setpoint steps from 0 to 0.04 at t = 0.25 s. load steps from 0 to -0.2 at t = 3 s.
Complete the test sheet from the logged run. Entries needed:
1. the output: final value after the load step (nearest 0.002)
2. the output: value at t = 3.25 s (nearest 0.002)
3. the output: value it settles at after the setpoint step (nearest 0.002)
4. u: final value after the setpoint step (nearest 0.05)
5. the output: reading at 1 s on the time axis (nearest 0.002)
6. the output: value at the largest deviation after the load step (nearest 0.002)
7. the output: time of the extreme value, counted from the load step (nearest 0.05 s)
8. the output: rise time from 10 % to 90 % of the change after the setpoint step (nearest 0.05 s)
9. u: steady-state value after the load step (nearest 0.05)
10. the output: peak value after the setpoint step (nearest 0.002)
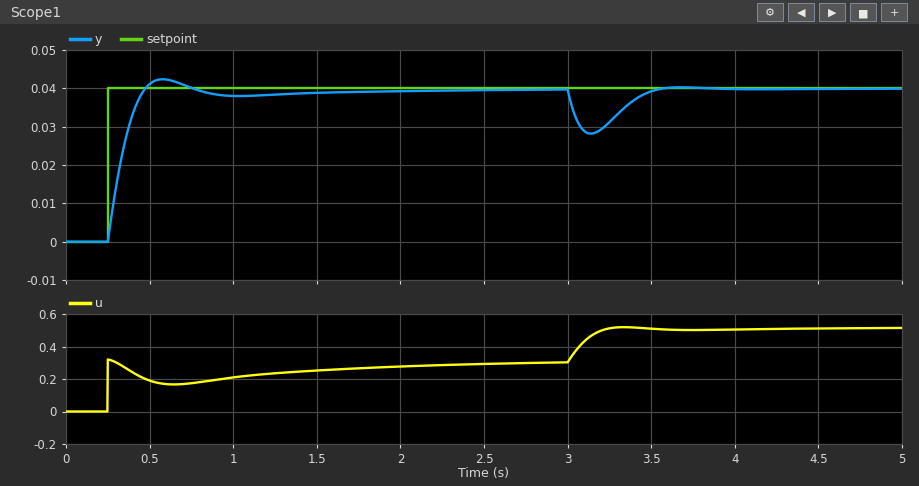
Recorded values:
0.040
0.032
0.040
0.30
0.038
0.028
0.15 s
0.15 s
0.50
0.042
